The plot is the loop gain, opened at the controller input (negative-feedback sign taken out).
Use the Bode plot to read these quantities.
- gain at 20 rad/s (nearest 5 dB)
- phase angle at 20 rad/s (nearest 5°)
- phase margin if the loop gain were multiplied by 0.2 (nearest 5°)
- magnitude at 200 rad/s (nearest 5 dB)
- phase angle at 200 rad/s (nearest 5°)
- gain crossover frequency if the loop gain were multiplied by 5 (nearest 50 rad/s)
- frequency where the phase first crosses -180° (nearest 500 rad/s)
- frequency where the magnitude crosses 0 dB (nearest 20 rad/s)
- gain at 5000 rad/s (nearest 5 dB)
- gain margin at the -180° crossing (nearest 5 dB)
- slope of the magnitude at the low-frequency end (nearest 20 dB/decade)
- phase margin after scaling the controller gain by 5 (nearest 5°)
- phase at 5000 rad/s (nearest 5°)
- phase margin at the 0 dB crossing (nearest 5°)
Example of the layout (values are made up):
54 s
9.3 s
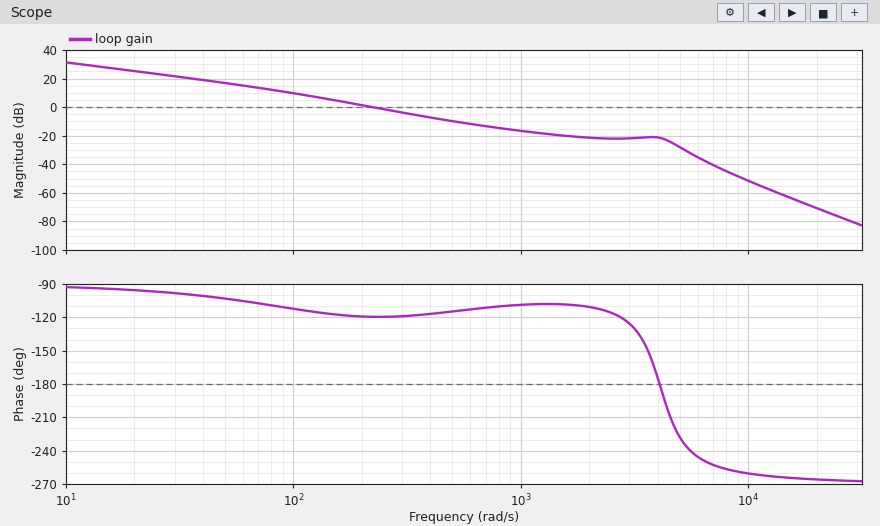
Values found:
25 dB
-95°
75°
0 dB
-120°
750 rad/s
4000 rad/s
220 rad/s
-30 dB
20 dB
-20 dB/decade
70°
-230°
60°
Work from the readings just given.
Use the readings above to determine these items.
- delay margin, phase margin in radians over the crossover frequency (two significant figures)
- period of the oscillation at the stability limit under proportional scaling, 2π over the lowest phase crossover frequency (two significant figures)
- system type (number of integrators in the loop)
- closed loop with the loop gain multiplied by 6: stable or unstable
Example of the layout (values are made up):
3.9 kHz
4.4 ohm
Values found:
0.0048 s
0.0016 s
1
stable
